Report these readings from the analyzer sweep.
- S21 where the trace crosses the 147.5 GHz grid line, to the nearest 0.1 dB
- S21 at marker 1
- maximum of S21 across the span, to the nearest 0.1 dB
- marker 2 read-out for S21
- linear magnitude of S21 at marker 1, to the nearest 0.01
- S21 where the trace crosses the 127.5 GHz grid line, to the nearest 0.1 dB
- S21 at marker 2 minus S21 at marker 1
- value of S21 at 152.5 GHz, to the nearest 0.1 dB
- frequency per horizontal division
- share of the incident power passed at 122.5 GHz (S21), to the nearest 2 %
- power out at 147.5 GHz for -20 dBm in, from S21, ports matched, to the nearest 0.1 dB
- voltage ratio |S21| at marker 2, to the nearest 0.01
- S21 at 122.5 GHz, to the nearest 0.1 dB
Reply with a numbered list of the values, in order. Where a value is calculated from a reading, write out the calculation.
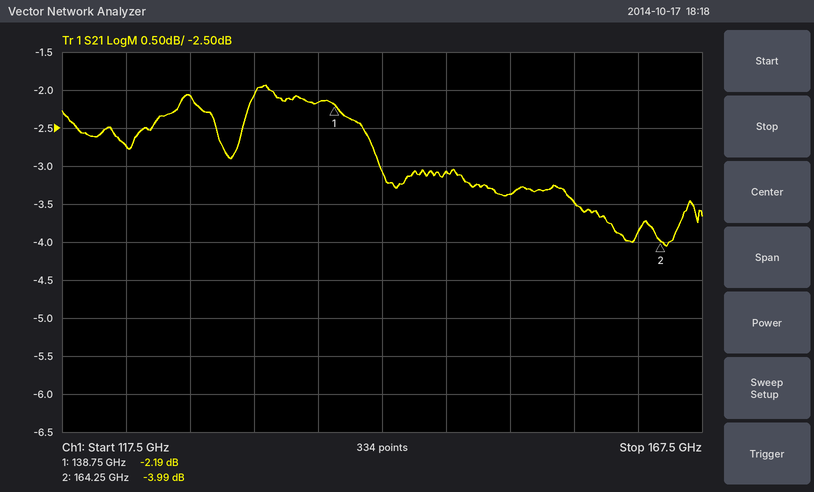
1. -3.1 dB
2. -2.19 dB
3. -1.9 dB
4. -3.99 dB
5. 10^(-2.19/20) ≈ 0.78
6. -2.1 dB
7. -3.99 − (-2.19) = -1.80 dB
8. -3.4 dB
9. 5 GHz
10. 10^(-2.7/10) ≈ 54 %
11. -20 dBm + (-3.1 dB) = -23.1 dBm
12. 10^(-3.99/20) ≈ 0.63
13. -2.7 dB
